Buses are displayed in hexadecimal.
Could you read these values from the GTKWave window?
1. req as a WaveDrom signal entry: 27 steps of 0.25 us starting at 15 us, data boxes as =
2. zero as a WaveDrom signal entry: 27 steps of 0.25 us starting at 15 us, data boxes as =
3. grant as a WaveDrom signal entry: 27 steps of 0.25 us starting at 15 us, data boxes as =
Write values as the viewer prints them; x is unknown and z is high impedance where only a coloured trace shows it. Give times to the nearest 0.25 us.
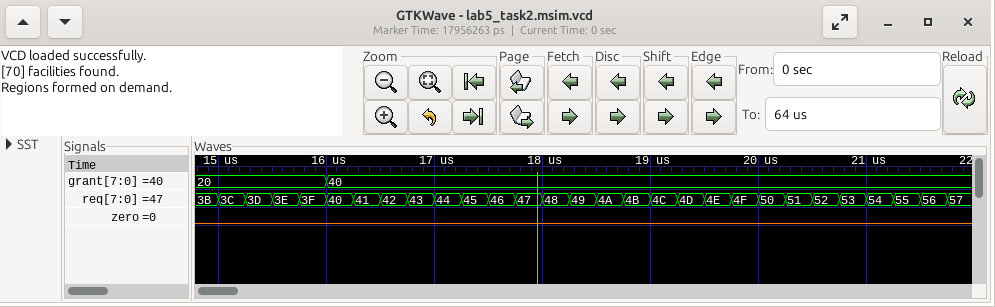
{name: 'req', wave: '===========================', data: '3C 3D 3E 3F 40 41 42 43 44 45 46 47 48 49 4A 4B 4C 4D 4E 4F 50 51 52 53 54 55 56'}
{name: 'zero', wave: '0..........................'}
{name: 'grant', wave: '=...=......................', data: '20 40'}
